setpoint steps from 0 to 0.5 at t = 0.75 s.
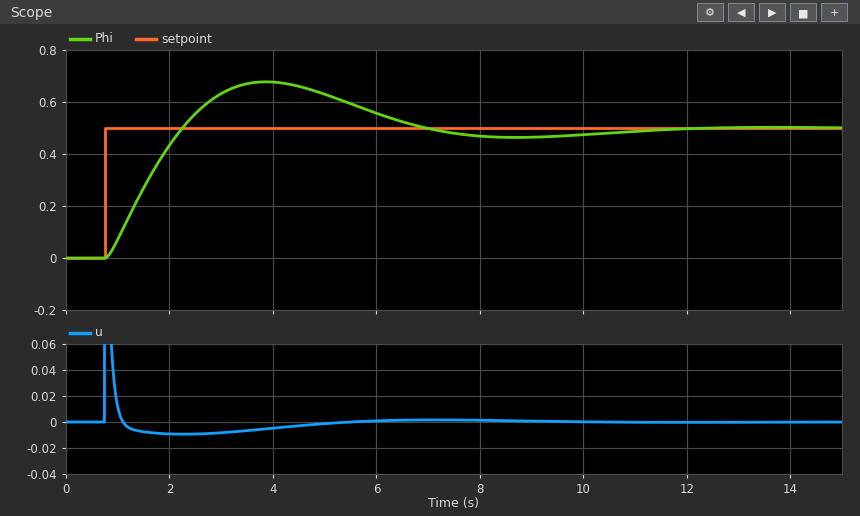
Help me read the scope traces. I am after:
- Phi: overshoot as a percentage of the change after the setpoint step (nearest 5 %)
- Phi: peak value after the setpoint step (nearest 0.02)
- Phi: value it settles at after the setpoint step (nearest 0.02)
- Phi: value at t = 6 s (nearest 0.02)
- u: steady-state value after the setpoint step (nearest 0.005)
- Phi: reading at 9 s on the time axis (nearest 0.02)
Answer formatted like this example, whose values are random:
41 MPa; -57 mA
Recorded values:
35 %; 0.68; 0.50; 0.56; 0.000; 0.46
